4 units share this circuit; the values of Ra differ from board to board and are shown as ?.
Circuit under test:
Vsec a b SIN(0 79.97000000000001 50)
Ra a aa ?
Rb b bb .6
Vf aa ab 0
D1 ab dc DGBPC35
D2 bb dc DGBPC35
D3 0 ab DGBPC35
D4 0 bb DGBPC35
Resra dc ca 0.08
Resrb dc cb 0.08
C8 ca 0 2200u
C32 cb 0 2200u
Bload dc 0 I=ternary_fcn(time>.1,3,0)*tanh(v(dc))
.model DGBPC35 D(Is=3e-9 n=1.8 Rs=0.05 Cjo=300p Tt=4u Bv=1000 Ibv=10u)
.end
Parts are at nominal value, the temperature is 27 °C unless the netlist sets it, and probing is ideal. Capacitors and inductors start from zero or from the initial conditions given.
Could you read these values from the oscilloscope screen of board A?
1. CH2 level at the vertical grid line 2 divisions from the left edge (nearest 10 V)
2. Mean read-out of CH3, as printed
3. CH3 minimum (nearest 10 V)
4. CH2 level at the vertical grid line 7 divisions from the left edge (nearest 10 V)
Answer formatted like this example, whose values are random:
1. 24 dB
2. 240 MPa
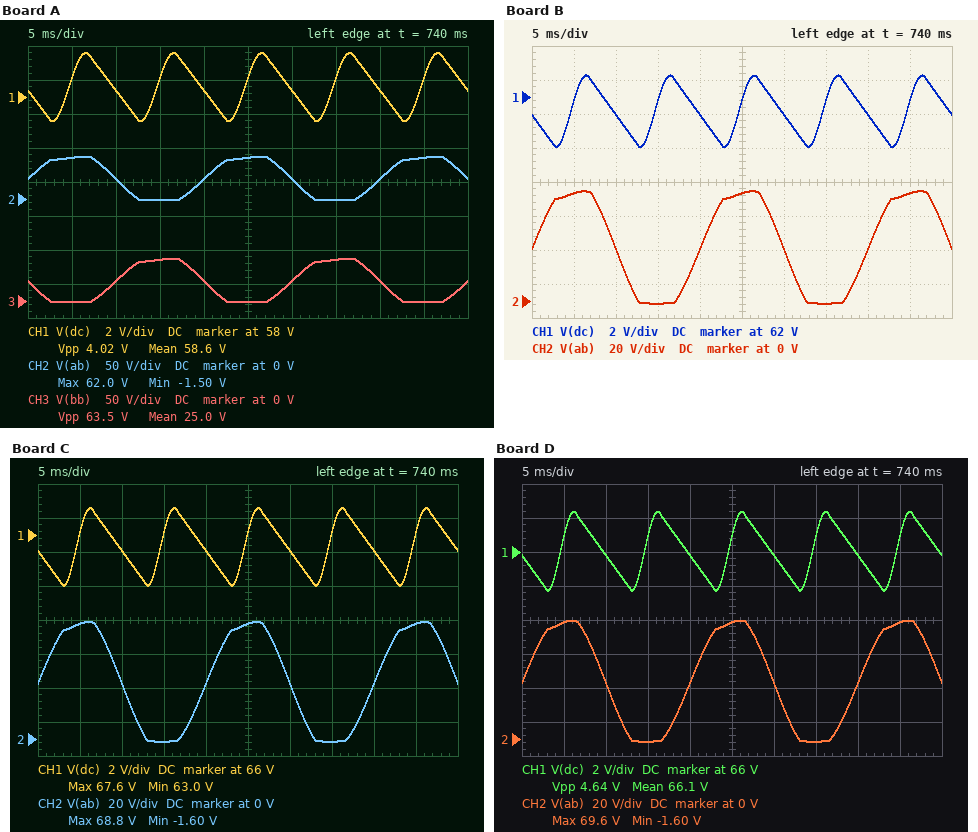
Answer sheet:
1. 30 V
2. 25.0 V
3. 0 V
4. 0 V
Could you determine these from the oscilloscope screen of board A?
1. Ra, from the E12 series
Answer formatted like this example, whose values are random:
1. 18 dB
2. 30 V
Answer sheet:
1. 1.2 Ω
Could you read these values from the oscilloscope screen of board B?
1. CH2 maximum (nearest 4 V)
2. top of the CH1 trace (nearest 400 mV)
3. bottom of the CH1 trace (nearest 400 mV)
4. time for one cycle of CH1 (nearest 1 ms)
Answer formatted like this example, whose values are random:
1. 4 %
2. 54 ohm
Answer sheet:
1. 64 V
2. 63.2 V
3. 59.2 V
4. 10 ms
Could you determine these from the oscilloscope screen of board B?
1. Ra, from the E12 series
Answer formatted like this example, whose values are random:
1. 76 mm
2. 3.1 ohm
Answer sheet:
1. 0.82 Ω
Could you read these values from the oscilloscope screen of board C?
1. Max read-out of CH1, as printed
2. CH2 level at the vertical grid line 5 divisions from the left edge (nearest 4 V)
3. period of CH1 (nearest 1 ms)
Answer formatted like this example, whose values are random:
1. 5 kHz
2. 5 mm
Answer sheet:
1. 67.6 V
2. 68 V
3. 10 ms
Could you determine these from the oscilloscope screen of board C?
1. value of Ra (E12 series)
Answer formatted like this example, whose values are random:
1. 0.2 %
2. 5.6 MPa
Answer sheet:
1. 0.27 Ω
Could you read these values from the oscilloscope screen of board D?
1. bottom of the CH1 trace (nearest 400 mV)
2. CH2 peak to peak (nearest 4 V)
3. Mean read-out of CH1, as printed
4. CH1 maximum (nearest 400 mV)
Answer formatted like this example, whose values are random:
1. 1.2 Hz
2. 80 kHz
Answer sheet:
1. 63.6 V
2. 72 V
3. 66.1 V
4. 68.4 V
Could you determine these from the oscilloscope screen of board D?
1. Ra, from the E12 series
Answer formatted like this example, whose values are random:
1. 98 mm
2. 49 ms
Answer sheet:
1. 0.18 Ω
